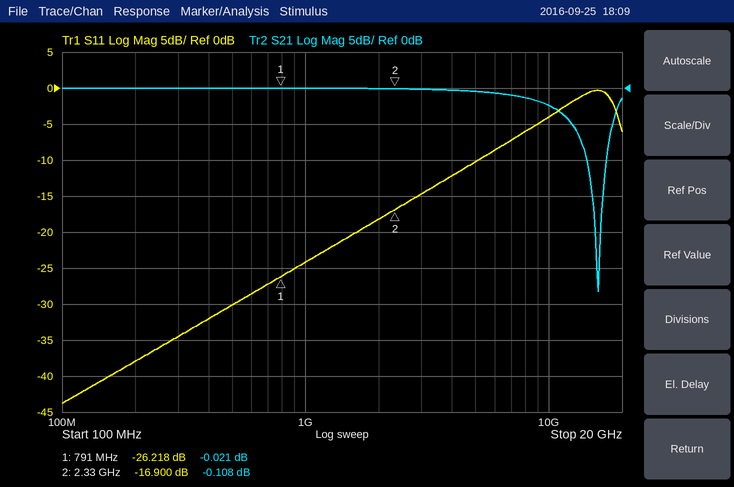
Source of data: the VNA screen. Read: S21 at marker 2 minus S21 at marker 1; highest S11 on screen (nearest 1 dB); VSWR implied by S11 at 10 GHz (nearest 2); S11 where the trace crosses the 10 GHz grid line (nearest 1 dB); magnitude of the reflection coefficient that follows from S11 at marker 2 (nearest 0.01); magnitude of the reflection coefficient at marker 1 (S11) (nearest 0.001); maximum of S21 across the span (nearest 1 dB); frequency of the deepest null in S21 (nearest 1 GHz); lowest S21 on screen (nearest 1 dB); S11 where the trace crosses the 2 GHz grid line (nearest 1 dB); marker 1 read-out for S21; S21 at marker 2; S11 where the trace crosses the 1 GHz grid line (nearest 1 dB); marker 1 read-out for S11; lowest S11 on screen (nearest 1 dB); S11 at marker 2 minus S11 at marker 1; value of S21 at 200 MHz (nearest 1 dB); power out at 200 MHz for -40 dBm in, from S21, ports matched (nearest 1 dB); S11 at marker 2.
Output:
-0.087 dB
0 dB
4
-4 dB
0.14
0.049
0 dB
16 GHz
-28 dB
-18 dB
-0.021 dB
-0.108 dB
-24 dB
-26.218 dB
-44 dB
9.318 dB
0 dB
-40 dBm
-16.900 dB
